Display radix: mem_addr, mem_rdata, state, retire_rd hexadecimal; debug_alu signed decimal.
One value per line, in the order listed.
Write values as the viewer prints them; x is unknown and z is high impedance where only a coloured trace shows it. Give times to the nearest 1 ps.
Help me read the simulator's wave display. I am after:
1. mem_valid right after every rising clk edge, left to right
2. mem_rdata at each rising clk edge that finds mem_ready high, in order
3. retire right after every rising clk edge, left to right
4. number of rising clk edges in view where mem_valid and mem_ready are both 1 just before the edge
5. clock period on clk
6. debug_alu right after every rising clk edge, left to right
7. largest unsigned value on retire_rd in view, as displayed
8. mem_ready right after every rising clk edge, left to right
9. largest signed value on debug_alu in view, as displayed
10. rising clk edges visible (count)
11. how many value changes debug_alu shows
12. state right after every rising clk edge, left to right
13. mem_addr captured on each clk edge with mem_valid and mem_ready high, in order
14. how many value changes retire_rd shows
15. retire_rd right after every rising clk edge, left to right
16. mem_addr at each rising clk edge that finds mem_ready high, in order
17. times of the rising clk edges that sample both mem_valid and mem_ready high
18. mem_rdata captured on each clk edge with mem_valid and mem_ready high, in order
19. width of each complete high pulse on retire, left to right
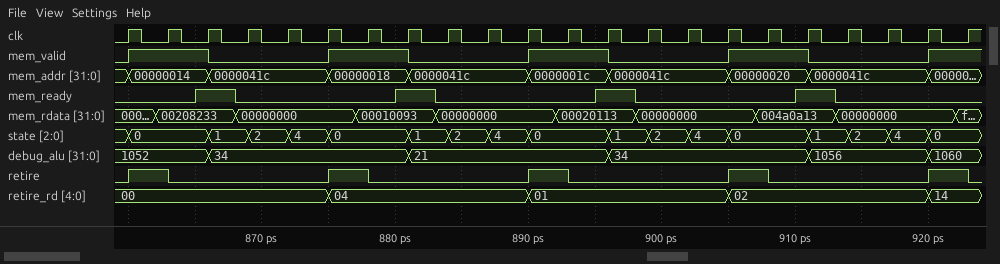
1 1 0 0 0 1 1 0 0 0 1 1 0 0 0 1 1 0 0 0 1 1
00208233, 00010093, 00020113, 004a0a13
1 0 0 0 0 1 0 0 0 0 1 0 0 0 0 1 0 0 0 0 1 0
4
3 ps
1052, 1052, 34, 34, 34, 34, 34, 21, 21, 21, 21, 21, 34, 34, 34, 34, 34, 1056, 1056, 1056, 1060, 1060
14
0 0 1 0 0 0 0 1 0 0 0 0 1 0 0 0 0 1 0 0 0 0
1060
22
5
0, 0, 1, 2, 4, 0, 0, 1, 2, 4, 0, 0, 1, 2, 4, 0, 0, 1, 2, 4, 0, 0
00000014, 00000018, 0000001c, 00000020
4
00, 00, 00, 00, 00, 04, 04, 04, 04, 04, 01, 01, 01, 01, 01, 02, 02, 02, 02, 02, 14, 14
00000014, 00000018, 0000001c, 00000020
866 ps, 881 ps, 896 ps, 911 ps
00208233, 00010093, 00020113, 004a0a13
3 ps, 3 ps, 3 ps, 3 ps, 3 ps
